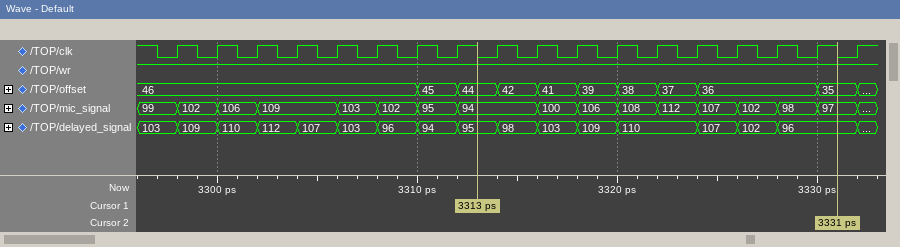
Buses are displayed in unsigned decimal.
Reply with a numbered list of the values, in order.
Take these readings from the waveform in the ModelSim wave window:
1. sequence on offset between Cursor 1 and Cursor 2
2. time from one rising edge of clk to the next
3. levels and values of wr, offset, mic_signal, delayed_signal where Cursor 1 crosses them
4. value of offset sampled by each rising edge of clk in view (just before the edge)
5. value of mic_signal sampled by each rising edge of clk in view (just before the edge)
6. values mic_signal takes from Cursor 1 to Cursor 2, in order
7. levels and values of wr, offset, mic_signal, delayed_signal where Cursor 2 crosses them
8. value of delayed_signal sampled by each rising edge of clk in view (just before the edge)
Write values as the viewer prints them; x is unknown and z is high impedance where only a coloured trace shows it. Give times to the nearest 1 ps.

1. 44, 42, 41, 39, 38, 37, 36, 35
2. 2 ps
3. wr=1, offset=44, mic_signal=94, delayed_signal=95
4. 46, 46, 46, 46, 46, 46, 46, 45, 44, 42, 41, 39, 38, 37, 36, 36, 36, 35
5. 99, 102, 106, 109, 109, 103, 102, 95, 94, 94, 100, 106, 108, 112, 107, 102, 98, 97
6. 94, 100, 106, 108, 112, 107, 102, 98, 97
7. wr=1, offset=35, mic_signal=97, delayed_signal=96
8. 103, 109, 110, 112, 107, 103, 96, 94, 95, 98, 103, 109, 110, 110, 107, 102, 96, 96
